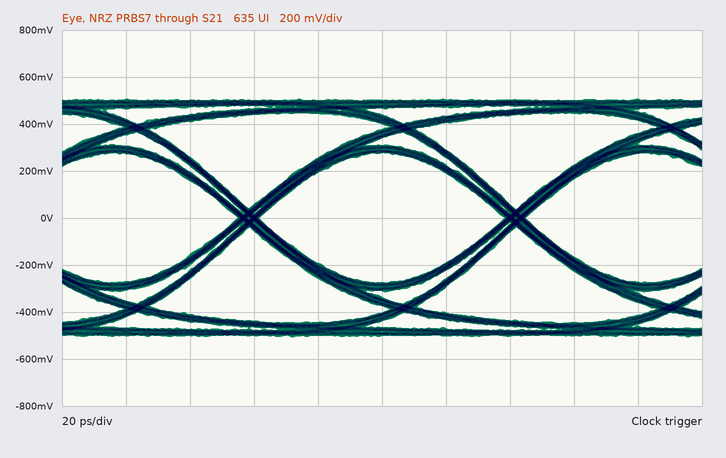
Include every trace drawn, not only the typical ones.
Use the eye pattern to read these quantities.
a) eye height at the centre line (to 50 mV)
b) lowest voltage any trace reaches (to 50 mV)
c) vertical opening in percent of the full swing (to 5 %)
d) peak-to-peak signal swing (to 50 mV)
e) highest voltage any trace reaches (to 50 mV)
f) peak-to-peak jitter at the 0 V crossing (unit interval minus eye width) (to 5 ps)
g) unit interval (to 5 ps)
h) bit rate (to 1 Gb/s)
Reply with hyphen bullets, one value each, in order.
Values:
- 550 mV
- -500 mV
- 55 %
- 1.00 V
- 500 mV
- 5 ps
- 85 ps
- 12 Gb/s
